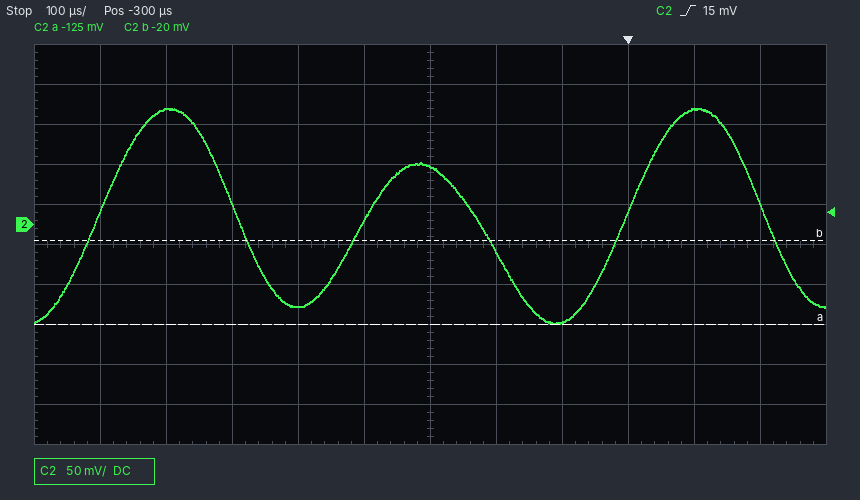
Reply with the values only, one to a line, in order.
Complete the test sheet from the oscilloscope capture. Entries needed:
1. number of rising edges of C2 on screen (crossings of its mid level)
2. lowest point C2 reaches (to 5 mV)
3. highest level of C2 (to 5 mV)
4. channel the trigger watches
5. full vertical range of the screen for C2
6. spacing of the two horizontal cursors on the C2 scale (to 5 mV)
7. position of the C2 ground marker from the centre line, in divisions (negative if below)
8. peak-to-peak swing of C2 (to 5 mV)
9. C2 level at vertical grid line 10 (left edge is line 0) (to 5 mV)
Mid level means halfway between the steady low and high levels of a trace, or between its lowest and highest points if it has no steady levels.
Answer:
3
-125 mV
145 mV
C2
500 mV
105 mV
+0.5 div
270 mV
145 mV
